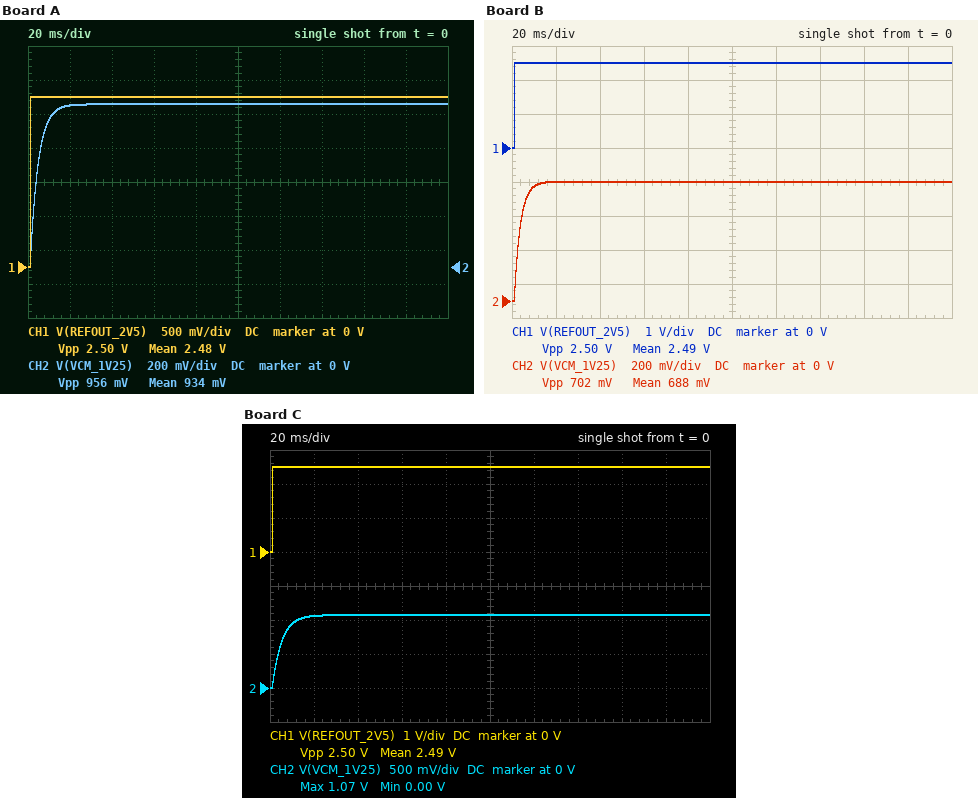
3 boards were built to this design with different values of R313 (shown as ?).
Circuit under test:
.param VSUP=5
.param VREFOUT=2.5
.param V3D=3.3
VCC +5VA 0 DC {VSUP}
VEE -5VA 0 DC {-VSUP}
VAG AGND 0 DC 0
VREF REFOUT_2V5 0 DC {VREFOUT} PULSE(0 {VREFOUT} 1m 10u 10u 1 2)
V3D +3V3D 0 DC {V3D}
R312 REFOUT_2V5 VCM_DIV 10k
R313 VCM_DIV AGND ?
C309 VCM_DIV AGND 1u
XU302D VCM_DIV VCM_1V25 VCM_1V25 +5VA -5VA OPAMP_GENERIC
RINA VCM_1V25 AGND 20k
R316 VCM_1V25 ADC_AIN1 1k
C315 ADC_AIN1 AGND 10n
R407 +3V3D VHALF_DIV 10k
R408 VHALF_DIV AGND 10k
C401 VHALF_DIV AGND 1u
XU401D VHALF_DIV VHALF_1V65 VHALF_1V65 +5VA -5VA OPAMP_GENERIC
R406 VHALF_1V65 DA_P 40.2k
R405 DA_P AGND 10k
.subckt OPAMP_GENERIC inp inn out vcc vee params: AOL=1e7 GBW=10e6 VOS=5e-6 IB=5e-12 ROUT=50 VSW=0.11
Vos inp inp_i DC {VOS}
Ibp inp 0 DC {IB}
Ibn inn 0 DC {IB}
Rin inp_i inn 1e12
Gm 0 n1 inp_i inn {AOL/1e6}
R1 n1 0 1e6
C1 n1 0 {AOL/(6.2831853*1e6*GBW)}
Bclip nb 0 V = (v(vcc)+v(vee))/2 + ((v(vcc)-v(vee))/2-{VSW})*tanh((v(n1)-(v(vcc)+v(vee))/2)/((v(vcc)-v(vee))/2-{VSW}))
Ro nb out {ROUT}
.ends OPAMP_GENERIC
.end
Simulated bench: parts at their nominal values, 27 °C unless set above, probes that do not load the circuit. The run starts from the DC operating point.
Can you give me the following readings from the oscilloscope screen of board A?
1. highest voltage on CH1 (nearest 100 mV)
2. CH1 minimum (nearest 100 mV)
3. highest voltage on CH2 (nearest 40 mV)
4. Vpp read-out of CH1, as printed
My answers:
2.5 V
0 V
960 mV
2.50 V
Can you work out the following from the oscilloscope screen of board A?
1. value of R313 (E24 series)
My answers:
6.2 kΩ
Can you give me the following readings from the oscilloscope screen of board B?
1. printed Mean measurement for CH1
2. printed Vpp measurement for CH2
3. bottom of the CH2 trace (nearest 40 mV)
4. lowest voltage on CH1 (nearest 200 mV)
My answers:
2.49 V
702 mV
0 V
0 V
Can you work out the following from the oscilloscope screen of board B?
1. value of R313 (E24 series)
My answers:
3.9 kΩ
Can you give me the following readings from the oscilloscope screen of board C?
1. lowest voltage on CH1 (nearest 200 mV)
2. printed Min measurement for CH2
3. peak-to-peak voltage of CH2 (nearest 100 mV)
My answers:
0 V
0.00 V
1.1 V
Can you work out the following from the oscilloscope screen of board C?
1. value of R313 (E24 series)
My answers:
7.5 kΩ
